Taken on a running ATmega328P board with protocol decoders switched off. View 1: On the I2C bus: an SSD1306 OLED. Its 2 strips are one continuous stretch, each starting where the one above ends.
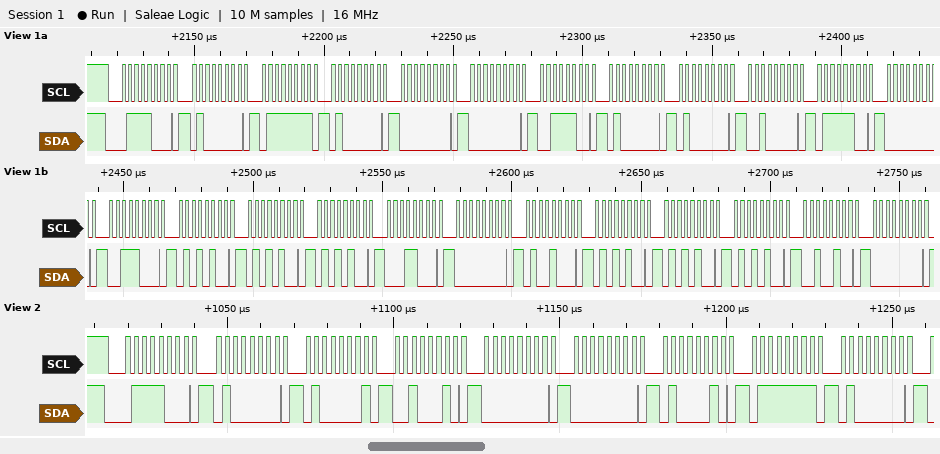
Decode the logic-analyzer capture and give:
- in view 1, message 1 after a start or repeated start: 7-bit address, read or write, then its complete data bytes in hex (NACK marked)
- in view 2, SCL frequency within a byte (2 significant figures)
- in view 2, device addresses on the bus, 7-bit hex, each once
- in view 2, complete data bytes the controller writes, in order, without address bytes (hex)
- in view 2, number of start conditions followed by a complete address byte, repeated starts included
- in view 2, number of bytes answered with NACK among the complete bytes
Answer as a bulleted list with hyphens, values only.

- 0x3C write: 40 7F 40 00 00 3C 40 40 20 7C 00 38 54 54 54 18 00 48 54 54 54 24 00
- 400 kHz
- 0x3C
- 40 41 22 00 00 42 7F 40
- 1
- 0
